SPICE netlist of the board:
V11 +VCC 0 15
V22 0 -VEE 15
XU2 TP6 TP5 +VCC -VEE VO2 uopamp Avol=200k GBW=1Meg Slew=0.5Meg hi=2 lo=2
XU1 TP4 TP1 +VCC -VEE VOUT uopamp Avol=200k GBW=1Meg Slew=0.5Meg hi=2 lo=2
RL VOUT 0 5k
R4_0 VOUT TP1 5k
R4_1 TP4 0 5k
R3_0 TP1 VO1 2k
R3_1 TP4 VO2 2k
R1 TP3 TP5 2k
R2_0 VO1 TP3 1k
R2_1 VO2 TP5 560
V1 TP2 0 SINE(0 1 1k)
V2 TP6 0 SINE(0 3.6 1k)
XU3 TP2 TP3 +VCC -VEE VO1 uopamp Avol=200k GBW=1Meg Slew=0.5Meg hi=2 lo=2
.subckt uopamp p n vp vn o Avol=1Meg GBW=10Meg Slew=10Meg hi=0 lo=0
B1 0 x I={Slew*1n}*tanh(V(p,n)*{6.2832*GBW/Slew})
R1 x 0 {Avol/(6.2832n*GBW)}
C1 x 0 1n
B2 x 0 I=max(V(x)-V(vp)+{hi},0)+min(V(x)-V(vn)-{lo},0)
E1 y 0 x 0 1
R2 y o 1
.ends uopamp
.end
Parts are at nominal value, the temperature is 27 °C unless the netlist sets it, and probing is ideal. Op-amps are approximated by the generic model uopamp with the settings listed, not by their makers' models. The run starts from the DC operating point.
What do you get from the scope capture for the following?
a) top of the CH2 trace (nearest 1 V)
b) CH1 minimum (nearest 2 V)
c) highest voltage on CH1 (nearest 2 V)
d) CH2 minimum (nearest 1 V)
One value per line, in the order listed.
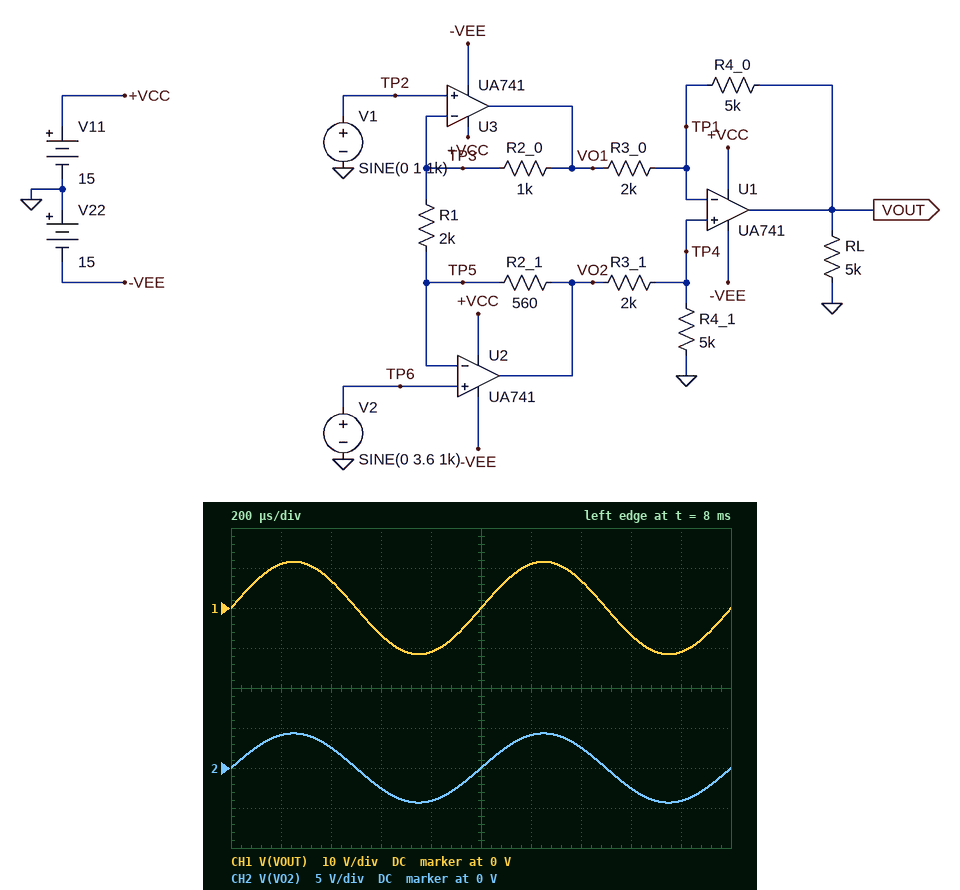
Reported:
4 V
-12 V
12 V
-4 V
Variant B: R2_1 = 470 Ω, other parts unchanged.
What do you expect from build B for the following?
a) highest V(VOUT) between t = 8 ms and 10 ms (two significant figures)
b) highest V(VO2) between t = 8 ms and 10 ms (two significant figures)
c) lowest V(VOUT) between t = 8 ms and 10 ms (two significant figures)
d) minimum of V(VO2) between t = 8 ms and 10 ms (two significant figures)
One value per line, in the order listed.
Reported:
11 V
4.2 V
-11 V
-4.2 V
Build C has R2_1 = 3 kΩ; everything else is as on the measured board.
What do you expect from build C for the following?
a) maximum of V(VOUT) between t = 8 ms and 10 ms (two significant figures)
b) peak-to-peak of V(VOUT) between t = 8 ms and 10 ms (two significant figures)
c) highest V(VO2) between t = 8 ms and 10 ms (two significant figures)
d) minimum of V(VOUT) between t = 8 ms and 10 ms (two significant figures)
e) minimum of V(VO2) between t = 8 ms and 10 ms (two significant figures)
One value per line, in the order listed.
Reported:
13 V
26 V
7.5 V
-13 V
-7.5 V
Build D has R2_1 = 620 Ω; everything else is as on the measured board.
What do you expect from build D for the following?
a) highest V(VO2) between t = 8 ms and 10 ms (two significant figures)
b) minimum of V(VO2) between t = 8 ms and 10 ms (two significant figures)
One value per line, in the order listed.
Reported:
4.4 V
-4.4 V
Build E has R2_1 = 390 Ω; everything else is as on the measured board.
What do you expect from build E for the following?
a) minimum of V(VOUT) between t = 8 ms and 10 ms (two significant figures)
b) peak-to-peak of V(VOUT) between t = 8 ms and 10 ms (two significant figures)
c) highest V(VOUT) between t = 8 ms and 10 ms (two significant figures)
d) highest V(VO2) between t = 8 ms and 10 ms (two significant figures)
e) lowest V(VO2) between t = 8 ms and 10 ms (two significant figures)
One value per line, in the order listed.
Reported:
-11 V
22 V
11 V
4.1 V
-4.1 V
